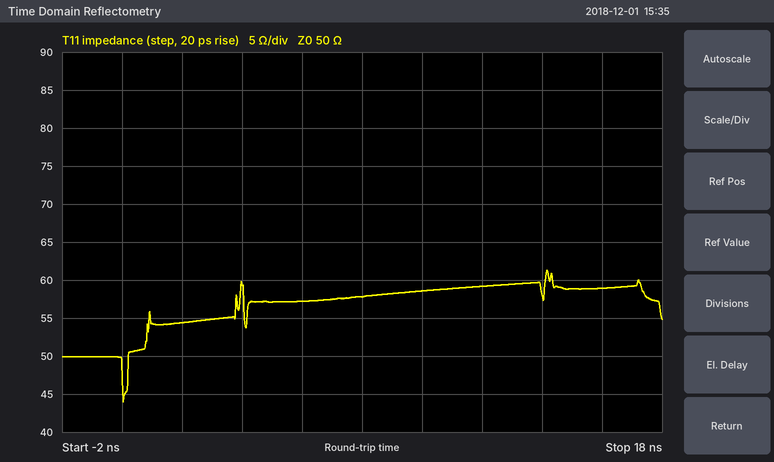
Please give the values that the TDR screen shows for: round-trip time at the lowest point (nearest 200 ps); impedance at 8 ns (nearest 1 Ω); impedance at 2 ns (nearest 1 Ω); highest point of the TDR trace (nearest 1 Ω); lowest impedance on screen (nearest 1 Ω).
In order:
0.0 ns
58 Ω
54 Ω
61 Ω
44 Ω
